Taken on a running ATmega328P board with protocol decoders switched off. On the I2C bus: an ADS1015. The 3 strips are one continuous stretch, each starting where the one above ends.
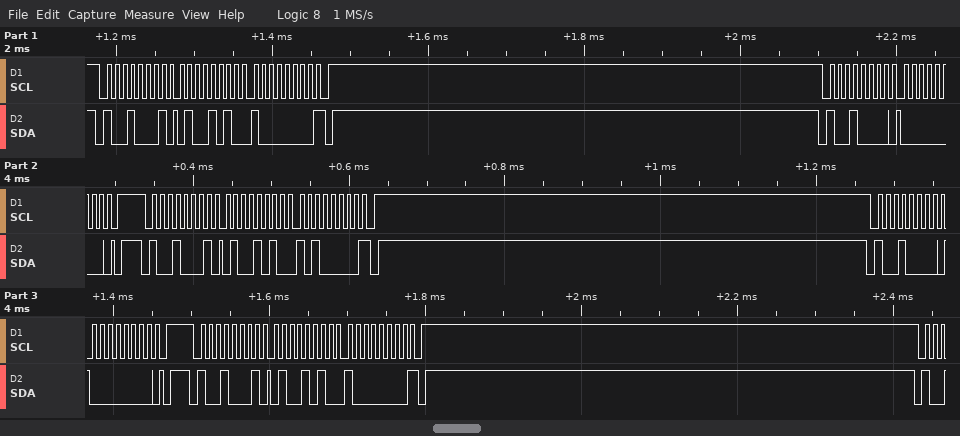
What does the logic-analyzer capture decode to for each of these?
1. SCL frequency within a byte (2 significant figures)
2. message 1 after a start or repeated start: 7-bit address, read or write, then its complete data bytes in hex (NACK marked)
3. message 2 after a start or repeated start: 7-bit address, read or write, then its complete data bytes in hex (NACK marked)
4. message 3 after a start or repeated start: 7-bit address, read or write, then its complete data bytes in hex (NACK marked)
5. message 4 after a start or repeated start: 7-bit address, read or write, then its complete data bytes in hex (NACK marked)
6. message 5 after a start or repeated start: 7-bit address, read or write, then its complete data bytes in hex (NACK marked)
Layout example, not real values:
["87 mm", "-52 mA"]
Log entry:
["100 kHz", "0x48 read: 4A 80 NACK", "0x48 write: 00", "0x48 read: 4A A0 NACK", "0x48 write: 00", "0x48 read: 4A 80 NACK"]
